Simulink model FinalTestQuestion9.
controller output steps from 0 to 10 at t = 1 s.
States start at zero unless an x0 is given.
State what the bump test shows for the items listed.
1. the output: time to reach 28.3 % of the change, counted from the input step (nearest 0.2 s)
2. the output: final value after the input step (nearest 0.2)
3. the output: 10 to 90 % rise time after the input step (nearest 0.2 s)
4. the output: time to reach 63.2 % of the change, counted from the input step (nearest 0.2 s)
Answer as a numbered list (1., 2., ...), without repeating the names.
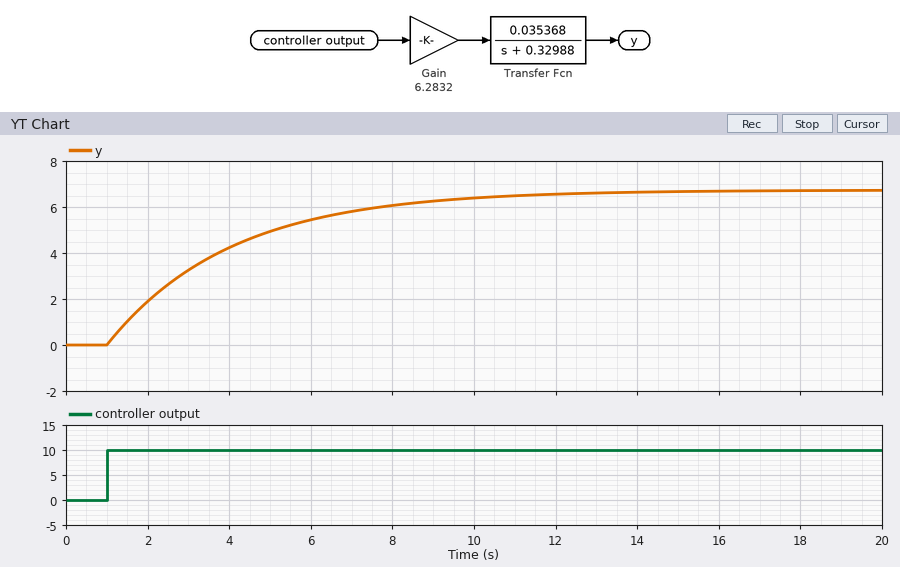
1. 1.0 s
2. 6.8
3. 6.6 s
4. 3.0 s
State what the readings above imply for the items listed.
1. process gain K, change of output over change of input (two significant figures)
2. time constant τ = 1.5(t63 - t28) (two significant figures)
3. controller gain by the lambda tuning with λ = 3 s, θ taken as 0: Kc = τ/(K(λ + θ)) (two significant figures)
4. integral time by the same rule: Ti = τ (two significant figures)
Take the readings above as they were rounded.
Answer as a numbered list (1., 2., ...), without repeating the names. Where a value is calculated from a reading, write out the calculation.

1. (6.8 - 0) / 10 = 0.68
2. 1.5 × (3 - 1) = 3.0 s
3. 3 / (0.68 × (3 + 0)) = 1.5
4. 3.0 s
